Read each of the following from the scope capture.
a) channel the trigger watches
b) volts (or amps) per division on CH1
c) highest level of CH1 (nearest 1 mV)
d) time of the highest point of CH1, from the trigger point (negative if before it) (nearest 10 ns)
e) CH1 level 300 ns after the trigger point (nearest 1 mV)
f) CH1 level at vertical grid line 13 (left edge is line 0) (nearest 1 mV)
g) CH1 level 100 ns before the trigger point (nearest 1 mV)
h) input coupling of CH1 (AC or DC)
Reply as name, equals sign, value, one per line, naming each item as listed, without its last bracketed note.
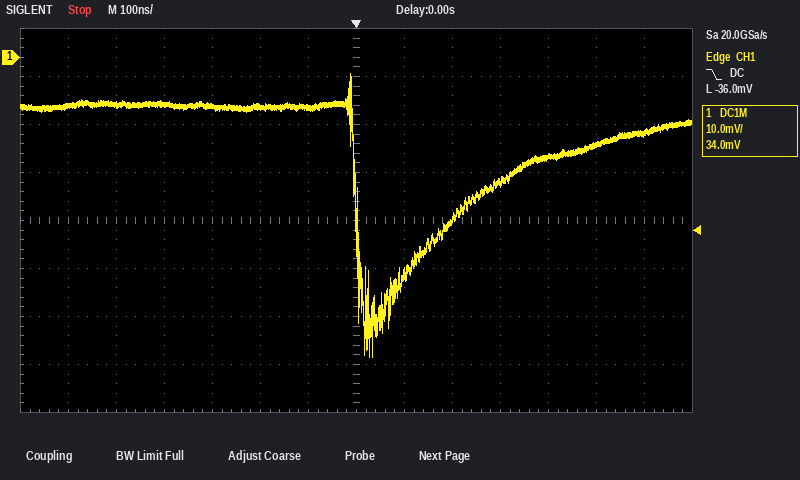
channel the trigger watches = CH1
volts (or amps) per division on CH1 = 10 mV
highest level of CH1 = -3 mV
time of the highest point of CH1, from the trigger point (negative if before it) = -10 ns
CH1 level 300 ns after the trigger point = -26 mV
CH1 level at vertical grid line 13 (left edge is line 0) = -16 mV
CH1 level 100 ns before the trigger point = -10 mV
input coupling of CH1 = DC
